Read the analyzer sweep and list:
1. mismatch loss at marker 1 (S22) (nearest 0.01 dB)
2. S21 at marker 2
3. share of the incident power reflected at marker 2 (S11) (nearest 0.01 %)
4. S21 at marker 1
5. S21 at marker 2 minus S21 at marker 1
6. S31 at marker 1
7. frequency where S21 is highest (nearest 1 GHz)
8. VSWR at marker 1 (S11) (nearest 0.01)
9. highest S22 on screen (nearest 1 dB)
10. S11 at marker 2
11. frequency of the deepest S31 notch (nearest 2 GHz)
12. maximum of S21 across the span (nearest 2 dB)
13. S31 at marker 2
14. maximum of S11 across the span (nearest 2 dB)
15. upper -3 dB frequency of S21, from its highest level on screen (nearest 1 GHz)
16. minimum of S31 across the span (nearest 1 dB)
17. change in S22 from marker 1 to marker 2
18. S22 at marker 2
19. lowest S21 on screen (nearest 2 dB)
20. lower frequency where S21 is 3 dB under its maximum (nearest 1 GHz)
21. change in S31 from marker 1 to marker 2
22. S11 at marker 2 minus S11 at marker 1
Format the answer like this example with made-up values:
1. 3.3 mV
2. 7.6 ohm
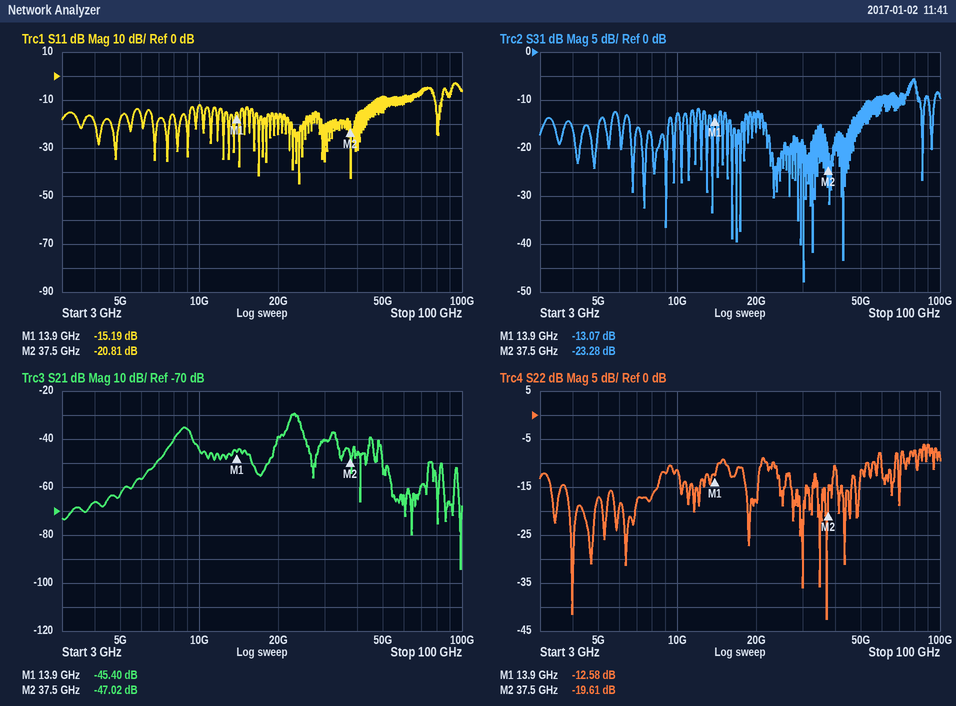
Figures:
1. 0.25 dB
2. -47.02 dB
3. 0.83 %
4. -45.40 dB
5. -1.62 dB
6. -13.07 dB
7. 23 GHz
8. 1.42
9. -6 dB
10. -20.81 dB
11. 30 GHz
12. -30 dB
13. -23.28 dB
14. -2 dB
15. 24 GHz
16. -48 dB
17. -7.03 dB
18. -19.61 dB
19. -94 dB
20. 22 GHz
21. -10.21 dB
22. -5.62 dB
